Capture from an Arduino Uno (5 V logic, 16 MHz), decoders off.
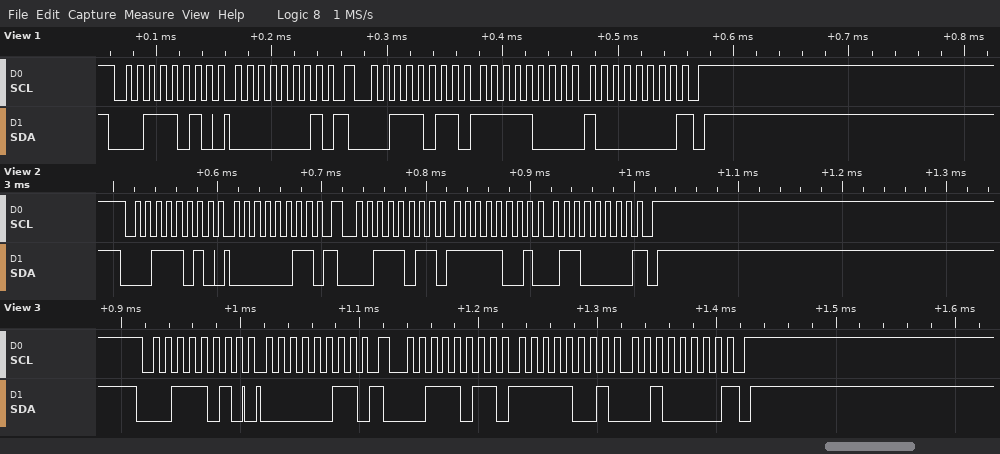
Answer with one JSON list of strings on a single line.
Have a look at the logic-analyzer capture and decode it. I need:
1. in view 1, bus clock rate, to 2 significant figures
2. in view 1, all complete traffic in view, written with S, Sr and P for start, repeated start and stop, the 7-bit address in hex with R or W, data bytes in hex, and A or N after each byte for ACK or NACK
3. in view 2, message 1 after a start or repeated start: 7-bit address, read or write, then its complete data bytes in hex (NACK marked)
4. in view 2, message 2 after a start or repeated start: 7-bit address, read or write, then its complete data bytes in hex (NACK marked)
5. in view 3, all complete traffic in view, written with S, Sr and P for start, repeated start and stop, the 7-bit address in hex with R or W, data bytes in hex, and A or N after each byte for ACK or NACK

["100 kHz", "S 1DW A 01 A Sr 1DR A F8 A 80 N P", "0x1D write: 03", "0x1D read: F9 60 NACK", "S 1DW A 03 A Sr 1DR A F9 A 20 N P"]
